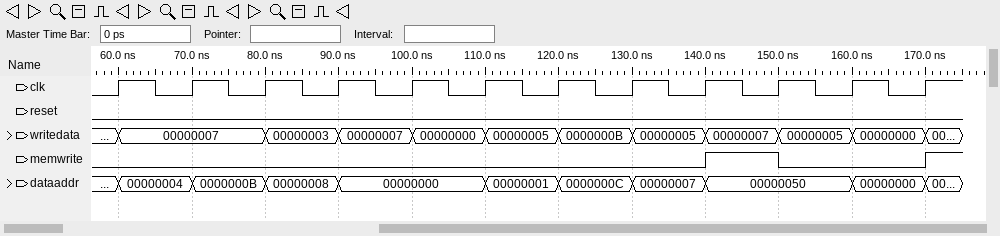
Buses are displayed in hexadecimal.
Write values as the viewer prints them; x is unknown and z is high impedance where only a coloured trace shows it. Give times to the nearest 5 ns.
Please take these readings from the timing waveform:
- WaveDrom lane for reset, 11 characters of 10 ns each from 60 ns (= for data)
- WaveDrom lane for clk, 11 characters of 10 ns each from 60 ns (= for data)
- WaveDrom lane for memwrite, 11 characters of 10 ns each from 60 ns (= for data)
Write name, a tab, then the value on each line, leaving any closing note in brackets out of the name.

WaveDrom lane for reset, 11 characters of 10 ns each from 60 ns	{name: 'reset', wave: '0..........'}
WaveDrom lane for clk, 11 characters of 10 ns each from 60 ns	{name: 'clk', wave: 'p..........'}
WaveDrom lane for memwrite, 11 characters of 10 ns each from 60 ns	{name: 'memwrite', wave: '0.......10.'}
